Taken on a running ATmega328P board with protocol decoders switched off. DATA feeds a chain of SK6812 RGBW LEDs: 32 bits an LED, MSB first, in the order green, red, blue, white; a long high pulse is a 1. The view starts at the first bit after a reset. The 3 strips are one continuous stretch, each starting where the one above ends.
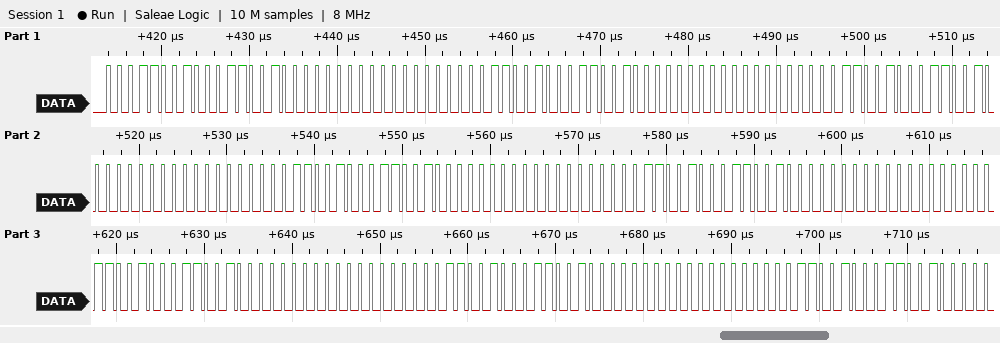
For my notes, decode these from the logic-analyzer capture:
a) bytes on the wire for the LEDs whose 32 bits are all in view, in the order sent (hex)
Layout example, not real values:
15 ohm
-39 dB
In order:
19 19 00 00 19 19 00 00 19 19 00 00 19 19 00 00 19 19 00 00 19 19 00 00 19 19 00 00
